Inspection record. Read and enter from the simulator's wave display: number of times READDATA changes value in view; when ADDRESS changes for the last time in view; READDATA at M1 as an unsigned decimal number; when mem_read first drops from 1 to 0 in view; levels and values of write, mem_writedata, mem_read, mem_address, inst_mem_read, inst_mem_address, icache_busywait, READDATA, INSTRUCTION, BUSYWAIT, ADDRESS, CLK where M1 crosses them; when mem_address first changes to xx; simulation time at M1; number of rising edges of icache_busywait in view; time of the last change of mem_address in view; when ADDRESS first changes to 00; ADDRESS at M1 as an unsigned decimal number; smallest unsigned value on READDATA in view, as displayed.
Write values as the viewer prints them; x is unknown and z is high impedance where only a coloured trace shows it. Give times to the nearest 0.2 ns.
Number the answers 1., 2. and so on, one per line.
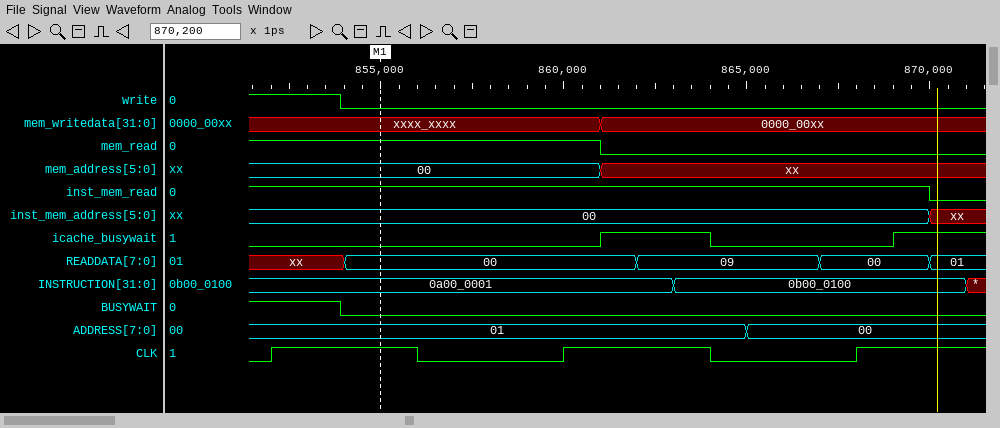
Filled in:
1. 4
2. 865 ns
3. 0
4. 861 ns
5. write=0, mem_writedata=xxxx_xxxx, mem_read=1, mem_address=00, inst_mem_read=1, inst_mem_address=00, icache_busywait=0, READDATA=00, INSTRUCTION=0a00_0001, BUSYWAIT=0, ADDRESS=01, CLK=1
6. 861 ns
7. 855 ns
8. 2
9. 861 ns
10. 865 ns
11. 1
12. 00
